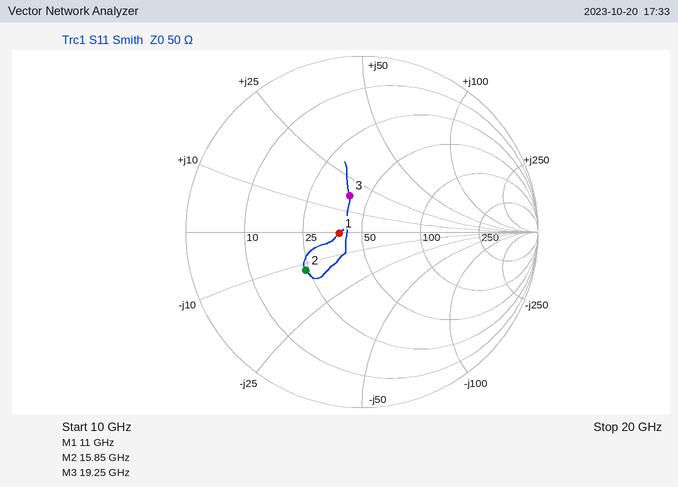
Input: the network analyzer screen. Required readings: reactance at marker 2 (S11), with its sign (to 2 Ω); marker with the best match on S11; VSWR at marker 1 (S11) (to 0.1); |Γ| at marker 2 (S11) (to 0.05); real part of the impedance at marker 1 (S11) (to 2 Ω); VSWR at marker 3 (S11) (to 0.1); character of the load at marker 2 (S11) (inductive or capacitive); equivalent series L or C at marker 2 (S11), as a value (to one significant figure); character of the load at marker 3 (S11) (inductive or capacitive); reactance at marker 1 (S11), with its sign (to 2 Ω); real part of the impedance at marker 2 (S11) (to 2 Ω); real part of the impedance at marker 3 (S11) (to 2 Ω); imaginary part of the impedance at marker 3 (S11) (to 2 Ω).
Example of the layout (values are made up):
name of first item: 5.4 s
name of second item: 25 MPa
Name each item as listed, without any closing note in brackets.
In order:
reactance at marker 2 (S11), with its sign: -12 Ω
marker with the best match on S11: marker 1
VSWR at marker 1 (S11): 1.3
|Γ| at marker 2 (S11): 0.40
real part of the impedance at marker 1 (S11): 38 Ω
VSWR at marker 3 (S11): 1.6
character of the load at marker 2 (S11): capacitive
equivalent series L or C at marker 2 (S11), as a value: 800 fF
character of the load at marker 3 (S11): inductive
reactance at marker 1 (S11), with its sign: 0 Ω
real part of the impedance at marker 2 (S11): 24 Ω
real part of the impedance at marker 3 (S11): 40 Ω
imaginary part of the impedance at marker 3 (S11): +18 Ω
